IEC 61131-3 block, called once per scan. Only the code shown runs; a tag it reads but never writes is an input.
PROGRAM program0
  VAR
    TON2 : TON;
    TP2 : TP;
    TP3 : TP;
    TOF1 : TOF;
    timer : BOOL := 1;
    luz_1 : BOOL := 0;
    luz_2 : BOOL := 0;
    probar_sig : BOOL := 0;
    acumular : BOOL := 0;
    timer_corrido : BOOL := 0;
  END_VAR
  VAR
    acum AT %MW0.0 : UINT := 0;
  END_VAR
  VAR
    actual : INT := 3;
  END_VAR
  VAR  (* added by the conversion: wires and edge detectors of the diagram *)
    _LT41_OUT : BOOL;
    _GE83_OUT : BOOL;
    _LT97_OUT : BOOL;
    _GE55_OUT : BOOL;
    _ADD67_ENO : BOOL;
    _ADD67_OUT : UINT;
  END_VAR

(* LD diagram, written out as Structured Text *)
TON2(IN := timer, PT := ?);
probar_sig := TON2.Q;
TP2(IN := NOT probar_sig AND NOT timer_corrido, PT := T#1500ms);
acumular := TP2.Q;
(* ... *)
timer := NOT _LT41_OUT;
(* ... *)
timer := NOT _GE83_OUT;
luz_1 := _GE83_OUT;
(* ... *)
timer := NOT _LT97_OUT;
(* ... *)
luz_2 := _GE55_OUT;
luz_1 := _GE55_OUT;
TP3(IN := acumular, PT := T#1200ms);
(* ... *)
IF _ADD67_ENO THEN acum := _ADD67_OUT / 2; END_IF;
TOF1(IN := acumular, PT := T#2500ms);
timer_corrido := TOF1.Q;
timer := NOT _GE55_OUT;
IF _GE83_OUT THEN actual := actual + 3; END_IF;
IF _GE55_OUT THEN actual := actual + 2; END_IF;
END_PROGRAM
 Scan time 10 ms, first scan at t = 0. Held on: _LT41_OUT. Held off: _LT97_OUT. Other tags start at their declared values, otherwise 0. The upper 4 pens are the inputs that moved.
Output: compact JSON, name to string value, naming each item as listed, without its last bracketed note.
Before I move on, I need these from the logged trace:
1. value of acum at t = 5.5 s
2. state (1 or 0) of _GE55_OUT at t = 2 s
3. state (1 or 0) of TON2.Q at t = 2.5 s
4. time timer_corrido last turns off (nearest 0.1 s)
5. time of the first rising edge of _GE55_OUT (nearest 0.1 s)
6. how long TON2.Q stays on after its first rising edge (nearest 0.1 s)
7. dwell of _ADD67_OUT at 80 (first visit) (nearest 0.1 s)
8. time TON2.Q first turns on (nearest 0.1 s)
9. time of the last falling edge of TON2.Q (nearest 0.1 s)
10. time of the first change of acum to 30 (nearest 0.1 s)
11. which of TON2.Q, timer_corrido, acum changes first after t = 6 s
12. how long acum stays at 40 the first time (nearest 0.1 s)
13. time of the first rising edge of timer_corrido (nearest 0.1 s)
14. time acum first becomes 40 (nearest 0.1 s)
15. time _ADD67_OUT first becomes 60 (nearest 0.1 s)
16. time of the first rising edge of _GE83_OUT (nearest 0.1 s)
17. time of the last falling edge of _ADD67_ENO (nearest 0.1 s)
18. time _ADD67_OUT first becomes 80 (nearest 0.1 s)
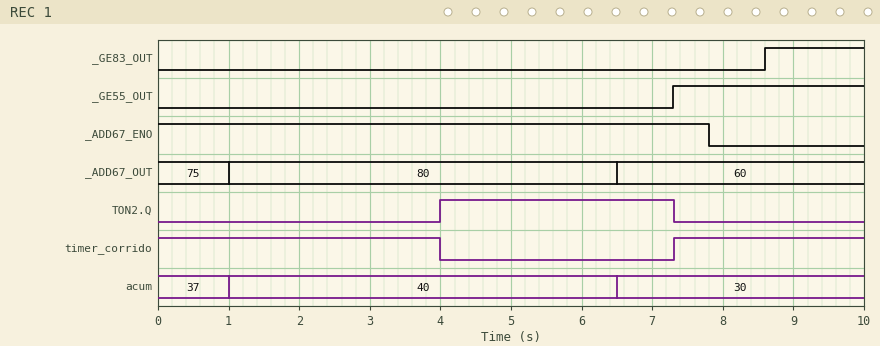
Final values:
{"value of acum at t = 5.5 s": "40", "state (1 or 0) of _GE55_OUT at t = 2 s": "0", "state (1 or 0) of TON2.Q at t = 2.5 s": "0", "time timer_corrido last turns off": "4.0 s", "time of the first rising edge of _GE55_OUT": "7.3 s", "how long TON2.Q stays on after its first rising edge": "3.3 s", "dwell of _ADD67_OUT at 80 (first visit)": "5.5 s", "time TON2.Q first turns on": "4.0 s", "time of the last falling edge of TON2.Q": "7.3 s", "time of the first change of acum to 30": "6.5 s", "which of TON2.Q, timer_corrido, acum changes first after t = 6 s": "acum", "how long acum stays at 40 the first time": "5.5 s", "time of the first rising edge of timer_corrido": "7.3 s", "time acum first becomes 40": "1.0 s", "time _ADD67_OUT first becomes 60": "6.5 s", "time of the first rising edge of _GE83_OUT": "8.6 s", "time of the last falling edge of _ADD67_ENO": "7.8 s", "time _ADD67_OUT first becomes 80": "1.0 s"}
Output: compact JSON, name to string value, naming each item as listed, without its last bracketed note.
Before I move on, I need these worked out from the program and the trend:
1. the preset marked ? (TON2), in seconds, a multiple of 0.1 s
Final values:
{"the preset marked ? (TON2), in seconds, a multiple of 0.1 s": "4.0 s"}
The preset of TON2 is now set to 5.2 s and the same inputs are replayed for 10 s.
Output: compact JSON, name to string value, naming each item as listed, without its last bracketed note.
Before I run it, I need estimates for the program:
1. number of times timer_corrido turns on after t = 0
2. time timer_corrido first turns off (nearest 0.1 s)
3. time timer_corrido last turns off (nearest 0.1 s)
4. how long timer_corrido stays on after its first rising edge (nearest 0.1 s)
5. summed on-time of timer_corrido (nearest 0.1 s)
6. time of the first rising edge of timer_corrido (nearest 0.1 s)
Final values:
{"number of times timer_corrido turns on after t = 0": "2", "time timer_corrido first turns off": "4.0 s", "time timer_corrido last turns off": "8.0 s", "how long timer_corrido stays on after its first rising edge": "4.0 s", "summed on-time of timer_corrido": "10.0 s", "time of the first rising edge of timer_corrido": "4.0 s"}
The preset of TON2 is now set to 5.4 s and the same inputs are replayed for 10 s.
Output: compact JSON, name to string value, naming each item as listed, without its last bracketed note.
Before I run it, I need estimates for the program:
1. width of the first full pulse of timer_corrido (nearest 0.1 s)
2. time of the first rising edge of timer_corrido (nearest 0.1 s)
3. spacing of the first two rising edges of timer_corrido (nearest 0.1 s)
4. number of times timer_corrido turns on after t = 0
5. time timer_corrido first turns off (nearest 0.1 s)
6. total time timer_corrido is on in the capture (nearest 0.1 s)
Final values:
{"width of the first full pulse of timer_corrido": "4.0 s", "time of the first rising edge of timer_corrido": "4.0 s", "spacing of the first two rising edges of timer_corrido": "4.0 s", "number of times timer_corrido turns on after t = 0": "2", "time timer_corrido first turns off": "4.0 s", "total time timer_corrido is on in the capture": "10.0 s"}
